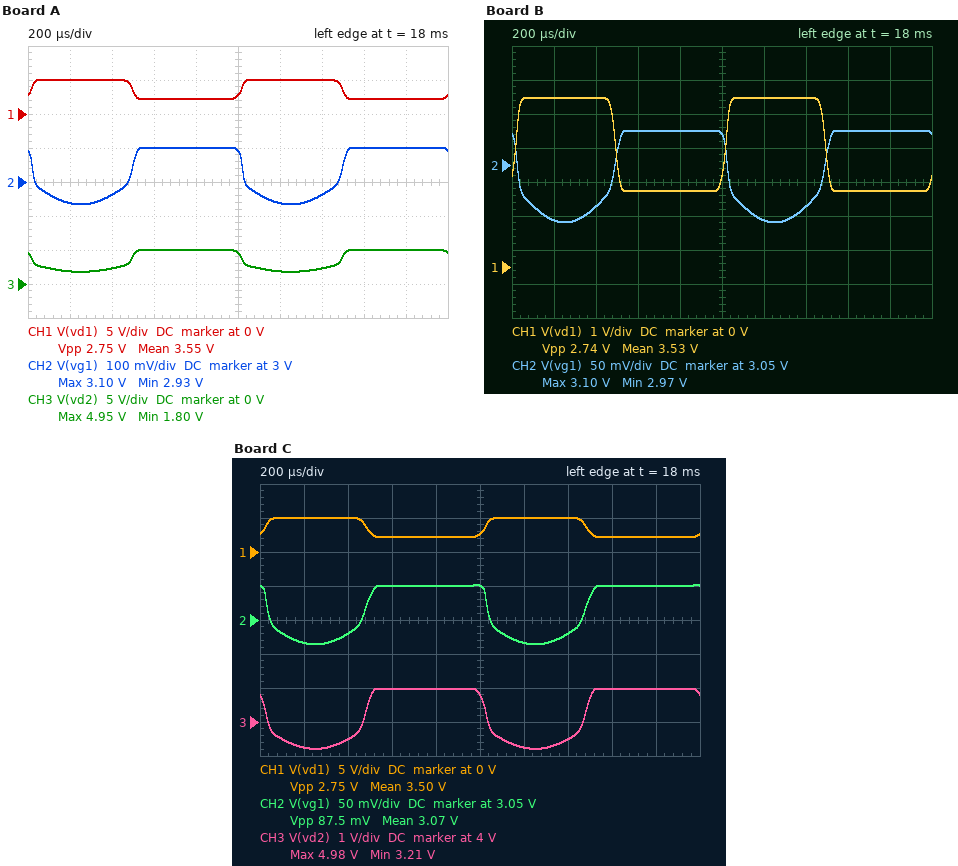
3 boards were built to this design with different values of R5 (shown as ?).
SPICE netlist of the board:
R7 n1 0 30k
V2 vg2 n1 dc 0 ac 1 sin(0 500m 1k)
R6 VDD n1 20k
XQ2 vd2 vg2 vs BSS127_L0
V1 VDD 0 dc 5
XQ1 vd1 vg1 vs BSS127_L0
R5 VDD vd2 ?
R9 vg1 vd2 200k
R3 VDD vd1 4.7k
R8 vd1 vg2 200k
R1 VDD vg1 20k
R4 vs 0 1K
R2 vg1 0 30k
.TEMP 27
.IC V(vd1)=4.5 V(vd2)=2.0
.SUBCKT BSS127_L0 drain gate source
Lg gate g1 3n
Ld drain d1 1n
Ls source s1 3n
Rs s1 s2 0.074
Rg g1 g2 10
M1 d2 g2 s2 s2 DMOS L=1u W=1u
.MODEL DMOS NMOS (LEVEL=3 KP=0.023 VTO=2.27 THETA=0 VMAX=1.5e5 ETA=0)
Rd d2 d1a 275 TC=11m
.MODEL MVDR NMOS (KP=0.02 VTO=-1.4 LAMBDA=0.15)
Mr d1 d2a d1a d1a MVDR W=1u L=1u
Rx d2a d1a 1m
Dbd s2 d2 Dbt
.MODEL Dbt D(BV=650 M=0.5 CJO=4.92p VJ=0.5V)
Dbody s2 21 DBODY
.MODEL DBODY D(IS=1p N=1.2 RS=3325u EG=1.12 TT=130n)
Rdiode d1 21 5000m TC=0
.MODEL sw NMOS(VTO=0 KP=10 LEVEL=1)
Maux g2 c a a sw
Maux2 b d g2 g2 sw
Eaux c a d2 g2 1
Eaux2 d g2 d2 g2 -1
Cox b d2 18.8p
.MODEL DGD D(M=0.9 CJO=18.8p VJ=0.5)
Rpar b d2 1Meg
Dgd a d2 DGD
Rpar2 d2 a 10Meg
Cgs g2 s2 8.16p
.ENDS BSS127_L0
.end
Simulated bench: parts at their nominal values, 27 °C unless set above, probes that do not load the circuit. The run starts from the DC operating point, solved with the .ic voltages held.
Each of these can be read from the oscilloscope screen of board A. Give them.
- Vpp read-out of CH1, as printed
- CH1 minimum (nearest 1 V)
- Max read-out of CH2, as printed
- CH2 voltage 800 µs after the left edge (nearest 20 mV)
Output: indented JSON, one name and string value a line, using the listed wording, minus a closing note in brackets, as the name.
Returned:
{
  "Vpp read-out of CH1, as printed": "2.75 V",
  "CH1 minimum": "2 V",
  "Max read-out of CH2, as printed": "3.10 V",
  "CH2 voltage 800 µs after the left edge": "3.10 V"
}
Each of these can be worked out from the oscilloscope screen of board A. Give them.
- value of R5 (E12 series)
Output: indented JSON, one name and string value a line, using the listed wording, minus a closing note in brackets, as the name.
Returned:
{
  "value of R5": "3.3 kΩ"
}
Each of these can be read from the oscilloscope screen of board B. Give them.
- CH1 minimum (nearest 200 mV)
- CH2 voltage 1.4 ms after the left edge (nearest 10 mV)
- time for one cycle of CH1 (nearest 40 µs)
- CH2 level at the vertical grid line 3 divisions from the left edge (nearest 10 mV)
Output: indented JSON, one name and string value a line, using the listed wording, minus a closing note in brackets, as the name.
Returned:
{
  "CH1 minimum": "2.2 V",
  "CH2 voltage 1.4 ms after the left edge": "2.99 V",
  "time for one cycle of CH1": "1.00 ms",
  "CH2 level at the vertical grid line 3 divisions from the left edge": "3.10 V"
}
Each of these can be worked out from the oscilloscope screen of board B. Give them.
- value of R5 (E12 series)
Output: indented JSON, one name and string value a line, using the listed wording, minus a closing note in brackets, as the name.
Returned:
{
  "value of R5": "2.7 kΩ"
}
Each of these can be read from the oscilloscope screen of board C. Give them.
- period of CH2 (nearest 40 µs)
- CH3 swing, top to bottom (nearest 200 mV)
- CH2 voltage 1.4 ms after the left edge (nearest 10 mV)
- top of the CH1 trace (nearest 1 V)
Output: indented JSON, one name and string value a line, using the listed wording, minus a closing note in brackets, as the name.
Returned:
{
  "period of CH2": "1.00 ms",
  "CH3 swing, top to bottom": "1.8 V",
  "CH2 voltage 1.4 ms after the left edge": "3.03 V",
  "top of the CH1 trace": "5 V"
}
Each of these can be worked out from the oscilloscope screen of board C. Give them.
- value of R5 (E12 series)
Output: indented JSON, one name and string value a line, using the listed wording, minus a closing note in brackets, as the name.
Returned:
{
  "value of R5": "1.8 kΩ"
}
